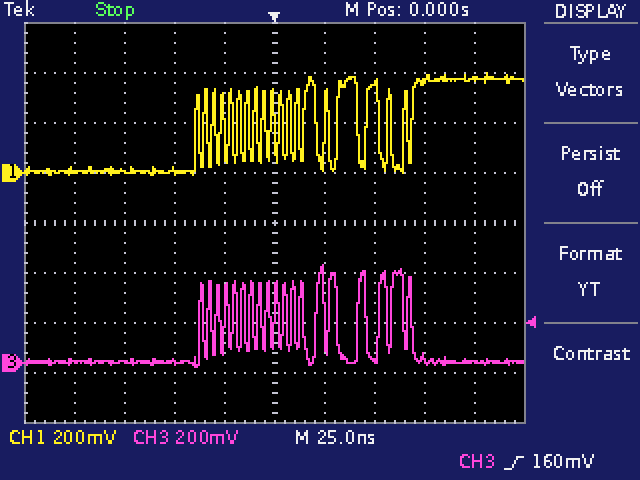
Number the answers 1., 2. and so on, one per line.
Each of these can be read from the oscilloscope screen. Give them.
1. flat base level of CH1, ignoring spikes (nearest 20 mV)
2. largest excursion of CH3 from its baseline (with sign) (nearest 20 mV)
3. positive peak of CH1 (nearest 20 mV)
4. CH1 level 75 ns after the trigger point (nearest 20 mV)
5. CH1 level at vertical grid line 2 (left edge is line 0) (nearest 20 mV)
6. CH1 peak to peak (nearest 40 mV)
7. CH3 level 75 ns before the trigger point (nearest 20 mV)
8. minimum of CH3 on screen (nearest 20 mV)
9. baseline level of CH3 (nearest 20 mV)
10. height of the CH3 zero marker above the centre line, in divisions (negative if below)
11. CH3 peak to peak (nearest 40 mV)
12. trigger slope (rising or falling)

1. 0 mV
2. +380 mV
3. 400 mV
4. 380 mV
5. 0 mV
6. 400 mV
7. 0 mV
8. -20 mV
9. 0 mV
10. -2.8 div
11. 400 mV
12. rising
